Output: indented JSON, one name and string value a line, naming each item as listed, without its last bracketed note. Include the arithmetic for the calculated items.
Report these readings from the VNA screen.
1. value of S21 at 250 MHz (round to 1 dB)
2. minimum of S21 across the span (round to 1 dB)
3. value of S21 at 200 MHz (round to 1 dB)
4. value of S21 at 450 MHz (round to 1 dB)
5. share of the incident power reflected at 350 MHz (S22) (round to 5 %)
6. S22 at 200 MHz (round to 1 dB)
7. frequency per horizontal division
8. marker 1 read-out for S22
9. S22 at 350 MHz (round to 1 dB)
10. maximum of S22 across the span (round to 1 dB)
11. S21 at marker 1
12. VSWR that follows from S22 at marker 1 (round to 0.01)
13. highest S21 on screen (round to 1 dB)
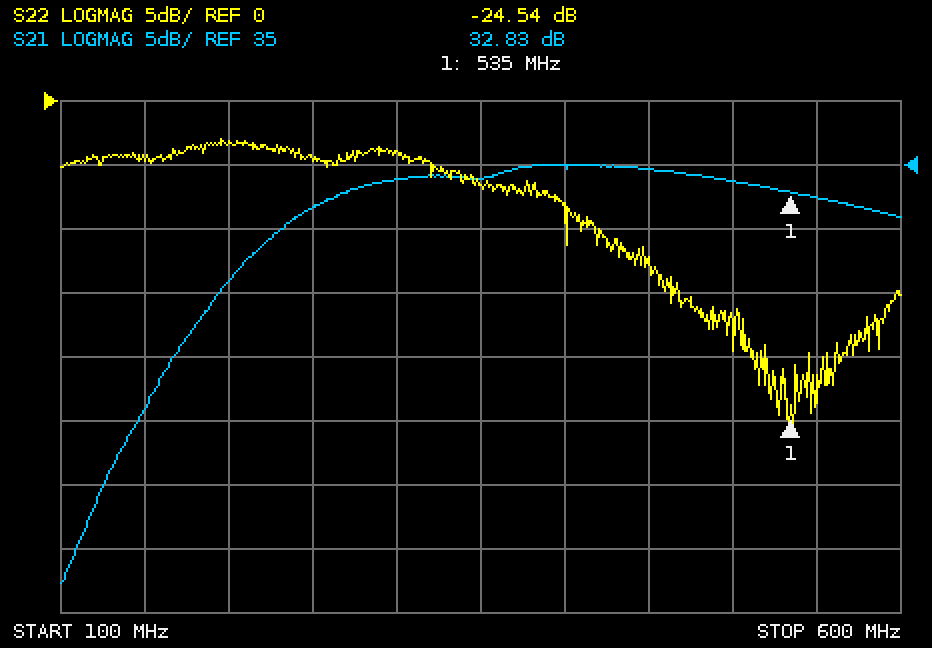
{
  "value of S21 at 250 MHz": "32 dB",
  "minimum of S21 across the span": "2 dB",
  "value of S21 at 200 MHz": "26 dB",
  "value of S21 at 450 MHz": "35 dB",
  "share of the incident power reflected at 350 MHz (S22)": "10^(-7/10) ≈ 20 %",
  "S22 at 200 MHz": "-3 dB",
  "frequency per horizontal division": "50 MHz",
  "marker 1 read-out for S22": "-24.54 dB",
  "S22 at 350 MHz": "-7 dB",
  "maximum of S22 across the span": "-3 dB",
  "S21 at marker 1": "32.83 dB",
  "VSWR that follows from S22 at marker 1": "(1 + 0.0593)/(1 − 0.0593) ≈ 1.13",
  "highest S21 on screen": "35 dB"
}
